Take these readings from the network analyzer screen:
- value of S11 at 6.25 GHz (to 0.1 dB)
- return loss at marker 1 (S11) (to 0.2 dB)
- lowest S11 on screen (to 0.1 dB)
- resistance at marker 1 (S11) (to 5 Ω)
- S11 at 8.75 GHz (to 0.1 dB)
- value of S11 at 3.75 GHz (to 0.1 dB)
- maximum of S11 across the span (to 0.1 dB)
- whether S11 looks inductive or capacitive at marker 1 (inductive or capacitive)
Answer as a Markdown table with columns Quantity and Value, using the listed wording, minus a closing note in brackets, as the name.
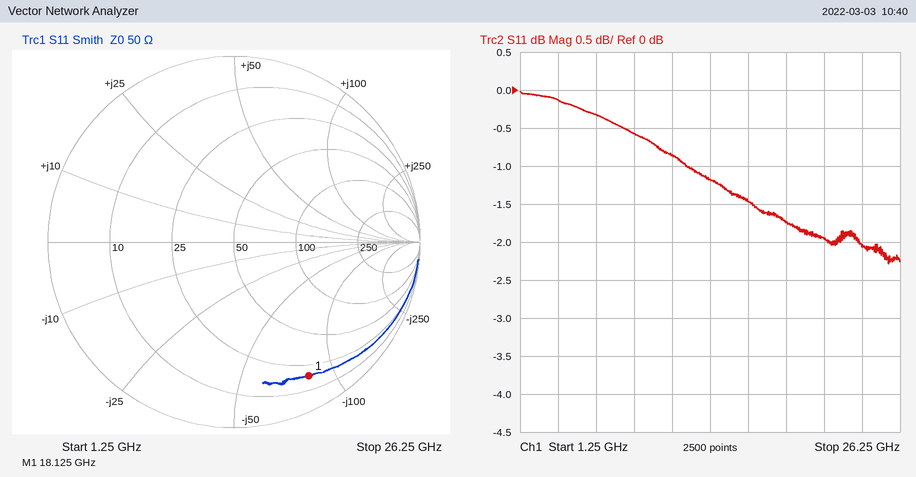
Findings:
| Quantity | Value |
|---|---|
| value of S11 at 6.25 GHz | -0.3 dB |
| return loss at marker 1 (S11) | 1.6 dB |
| lowest S11 on screen | -2.3 dB |
| resistance at marker 1 (S11) | 20 Ω |
| S11 at 8.75 GHz | -0.6 dB |
| value of S11 at 3.75 GHz | -0.1 dB |
| maximum of S11 across the span | 0.0 dB |
| whether S11 looks inductive or capacitive at marker 1 | capacitive |
